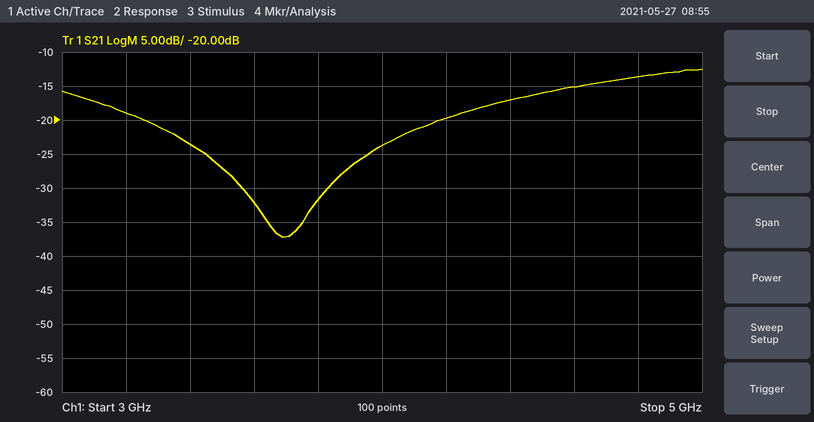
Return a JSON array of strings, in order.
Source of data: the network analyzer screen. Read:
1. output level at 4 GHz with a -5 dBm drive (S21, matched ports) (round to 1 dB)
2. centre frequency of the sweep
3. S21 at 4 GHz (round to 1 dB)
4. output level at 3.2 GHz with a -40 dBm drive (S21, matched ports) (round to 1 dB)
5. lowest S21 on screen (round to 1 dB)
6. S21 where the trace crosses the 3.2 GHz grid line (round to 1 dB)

["-29 dBm", "4 GHz", "-24 dB", "-59 dBm", "-37 dB", "-19 dB"]
